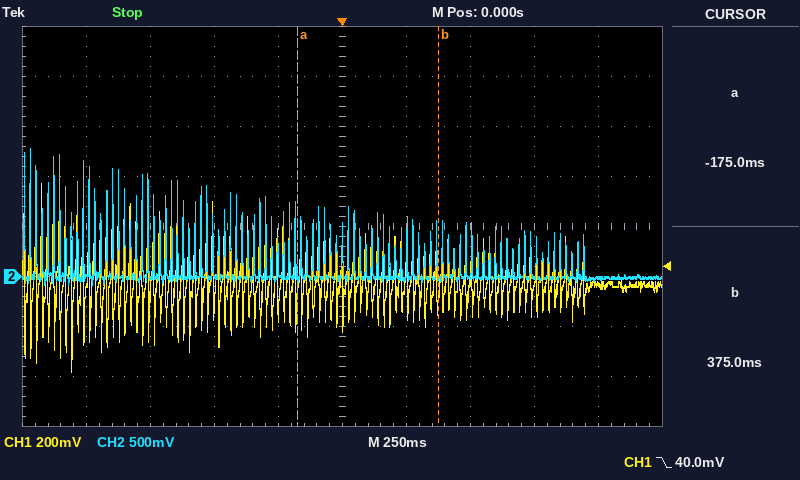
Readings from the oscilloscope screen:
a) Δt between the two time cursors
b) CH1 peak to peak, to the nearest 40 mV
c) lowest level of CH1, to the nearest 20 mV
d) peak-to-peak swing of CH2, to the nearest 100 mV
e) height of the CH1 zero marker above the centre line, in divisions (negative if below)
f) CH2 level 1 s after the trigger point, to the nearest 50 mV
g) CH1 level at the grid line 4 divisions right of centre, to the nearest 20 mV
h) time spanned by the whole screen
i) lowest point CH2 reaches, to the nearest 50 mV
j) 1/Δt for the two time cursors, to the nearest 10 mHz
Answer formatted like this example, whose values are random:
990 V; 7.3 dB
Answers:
550 ms; 760 mV; -380 mV; 1.40 V; -1.0 div; 0 mV; -40 mV; 2.5 s; -100 mV; 1.82 Hz
